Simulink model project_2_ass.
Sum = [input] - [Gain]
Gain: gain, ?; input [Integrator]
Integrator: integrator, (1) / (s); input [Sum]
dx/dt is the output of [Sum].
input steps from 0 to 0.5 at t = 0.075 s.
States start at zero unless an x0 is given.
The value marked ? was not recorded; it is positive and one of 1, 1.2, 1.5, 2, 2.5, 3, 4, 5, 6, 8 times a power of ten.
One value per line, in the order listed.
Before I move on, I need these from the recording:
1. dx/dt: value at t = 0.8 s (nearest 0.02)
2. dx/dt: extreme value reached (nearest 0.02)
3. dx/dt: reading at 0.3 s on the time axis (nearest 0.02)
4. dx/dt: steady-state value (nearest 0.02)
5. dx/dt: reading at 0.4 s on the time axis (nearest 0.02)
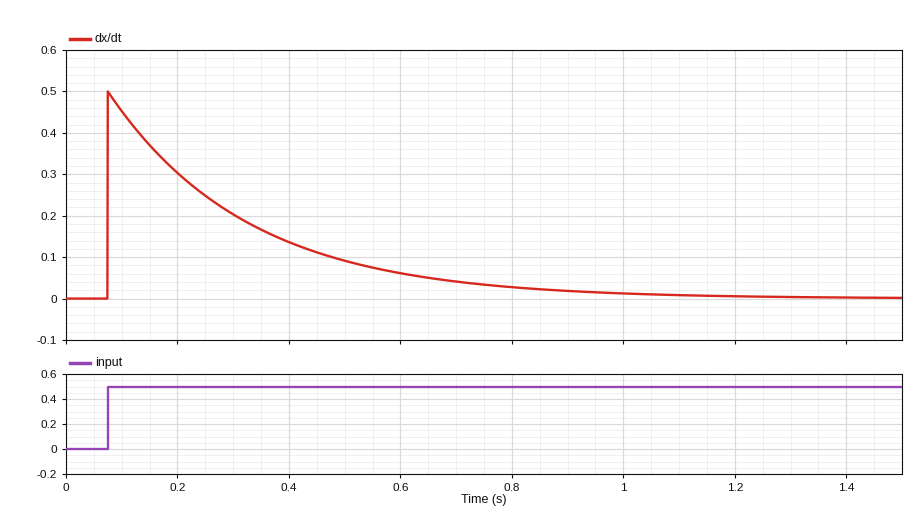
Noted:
0.02
0.50
0.20
0.00
0.14
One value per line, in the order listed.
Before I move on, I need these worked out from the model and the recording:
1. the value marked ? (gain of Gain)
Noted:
4
